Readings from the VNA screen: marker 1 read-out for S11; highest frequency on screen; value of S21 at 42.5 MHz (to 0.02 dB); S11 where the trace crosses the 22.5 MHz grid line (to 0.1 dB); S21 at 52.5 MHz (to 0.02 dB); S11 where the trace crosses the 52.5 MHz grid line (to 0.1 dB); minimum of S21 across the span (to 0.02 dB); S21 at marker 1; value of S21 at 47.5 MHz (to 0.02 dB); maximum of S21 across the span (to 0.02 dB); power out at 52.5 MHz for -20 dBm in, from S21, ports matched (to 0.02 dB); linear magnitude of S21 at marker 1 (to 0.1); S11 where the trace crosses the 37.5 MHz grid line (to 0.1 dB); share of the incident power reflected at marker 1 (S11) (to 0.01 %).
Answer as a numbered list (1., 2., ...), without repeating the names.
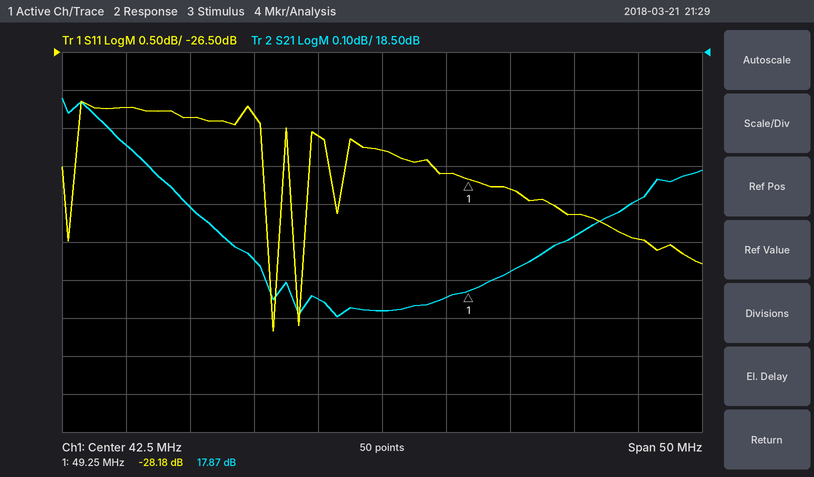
1. -28.18 dB
2. 67.5 MHz
3. 17.82 dB
4. -27.2 dB
5. 17.92 dB
6. -28.3 dB
7. 17.80 dB
8. 17.87 dB
9. 17.86 dB
10. 18.38 dB
11. -2.08 dBm
12. 7.8
13. -27.6 dB
14. 0.15 %
